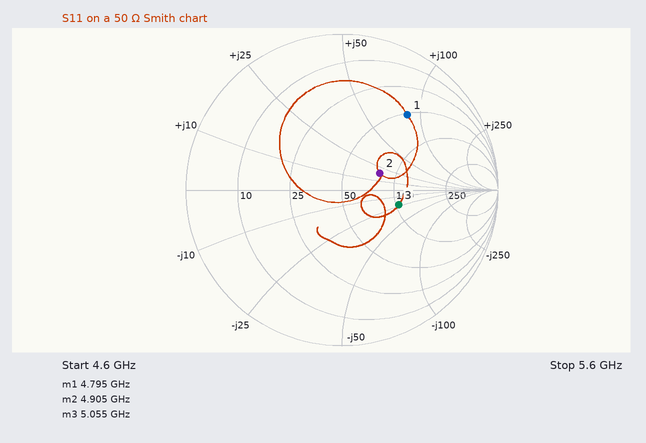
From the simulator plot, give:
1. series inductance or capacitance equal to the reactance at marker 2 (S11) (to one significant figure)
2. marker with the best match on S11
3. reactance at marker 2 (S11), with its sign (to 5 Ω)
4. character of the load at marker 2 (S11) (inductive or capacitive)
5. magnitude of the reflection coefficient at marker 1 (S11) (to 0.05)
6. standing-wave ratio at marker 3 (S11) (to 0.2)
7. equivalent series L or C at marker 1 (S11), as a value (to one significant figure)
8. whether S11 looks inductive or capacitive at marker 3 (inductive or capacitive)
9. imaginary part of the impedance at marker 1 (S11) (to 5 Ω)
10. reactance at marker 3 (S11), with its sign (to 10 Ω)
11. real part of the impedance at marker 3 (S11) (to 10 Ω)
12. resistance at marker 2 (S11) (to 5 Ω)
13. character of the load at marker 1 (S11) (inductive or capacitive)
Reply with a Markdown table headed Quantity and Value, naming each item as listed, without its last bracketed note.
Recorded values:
| Quantity | Value |
|---|---|
| series inductance or capacitance equal to the reactance at marker 2 (S11) | 600 pH |
| marker with the best match on S11 | marker 2 |
| reactance at marker 2 (S11), with its sign | +20 Ω |
| character of the load at marker 2 (S11) | inductive |
| magnitude of the reflection coefficient at marker 1 (S11) | 0.65 |
| standing-wave ratio at marker 3 (S11) | 2.2 |
| equivalent series L or C at marker 1 (S11), as a value | 3 nH |
| whether S11 looks inductive or capacitive at marker 3 | capacitive |
| imaginary part of the impedance at marker 1 (S11) | +85 Ω |
| reactance at marker 3 (S11), with its sign | -20 Ω |
| real part of the impedance at marker 3 (S11) | 100 Ω |
| resistance at marker 2 (S11) | 80 Ω |
| character of the load at marker 1 (S11) | inductive |
